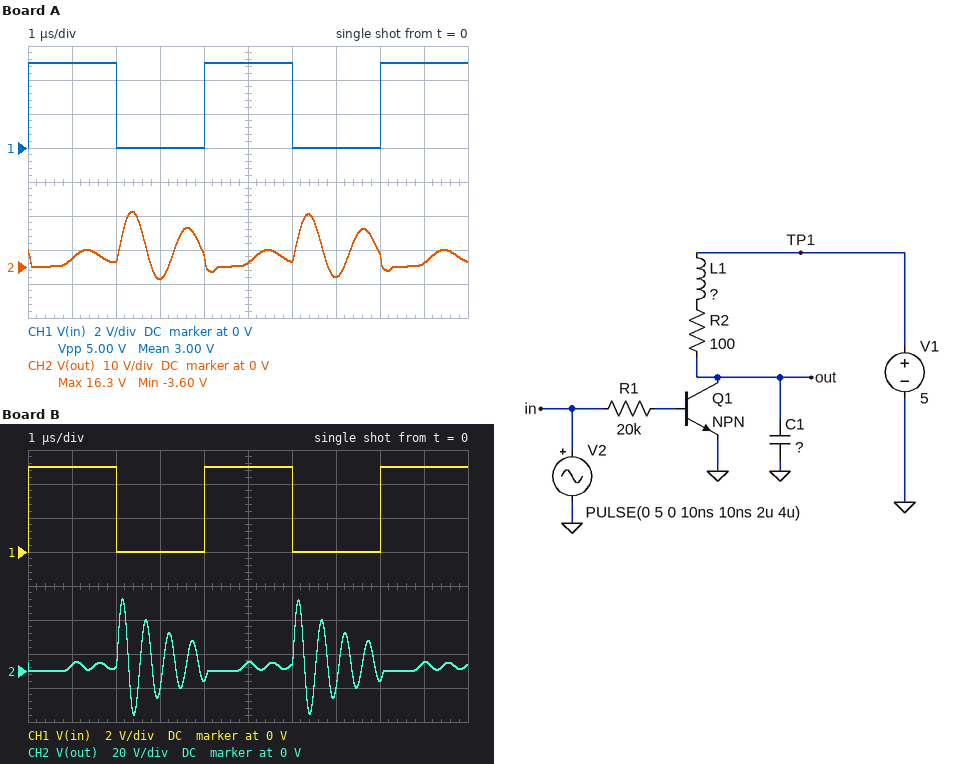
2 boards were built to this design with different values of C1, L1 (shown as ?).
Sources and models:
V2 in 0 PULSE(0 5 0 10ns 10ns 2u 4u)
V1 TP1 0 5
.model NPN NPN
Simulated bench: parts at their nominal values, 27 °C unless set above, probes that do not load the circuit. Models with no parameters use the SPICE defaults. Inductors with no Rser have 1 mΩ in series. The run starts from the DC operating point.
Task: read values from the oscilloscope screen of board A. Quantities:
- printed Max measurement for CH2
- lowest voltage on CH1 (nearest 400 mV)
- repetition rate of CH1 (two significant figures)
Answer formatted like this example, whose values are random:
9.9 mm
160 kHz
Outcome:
16.3 V
0 V
250 kHz
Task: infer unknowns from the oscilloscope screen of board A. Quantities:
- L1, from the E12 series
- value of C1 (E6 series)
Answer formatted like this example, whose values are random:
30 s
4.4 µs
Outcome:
120 µH
330 pF
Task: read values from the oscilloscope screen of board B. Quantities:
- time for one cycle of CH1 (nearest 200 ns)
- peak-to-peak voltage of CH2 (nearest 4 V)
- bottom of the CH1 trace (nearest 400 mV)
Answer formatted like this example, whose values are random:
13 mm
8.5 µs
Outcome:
4.0 µs
68 V
0 V
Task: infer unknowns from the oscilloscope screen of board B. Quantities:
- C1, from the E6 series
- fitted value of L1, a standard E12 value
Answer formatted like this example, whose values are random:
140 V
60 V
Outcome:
47 pF
150 µH
